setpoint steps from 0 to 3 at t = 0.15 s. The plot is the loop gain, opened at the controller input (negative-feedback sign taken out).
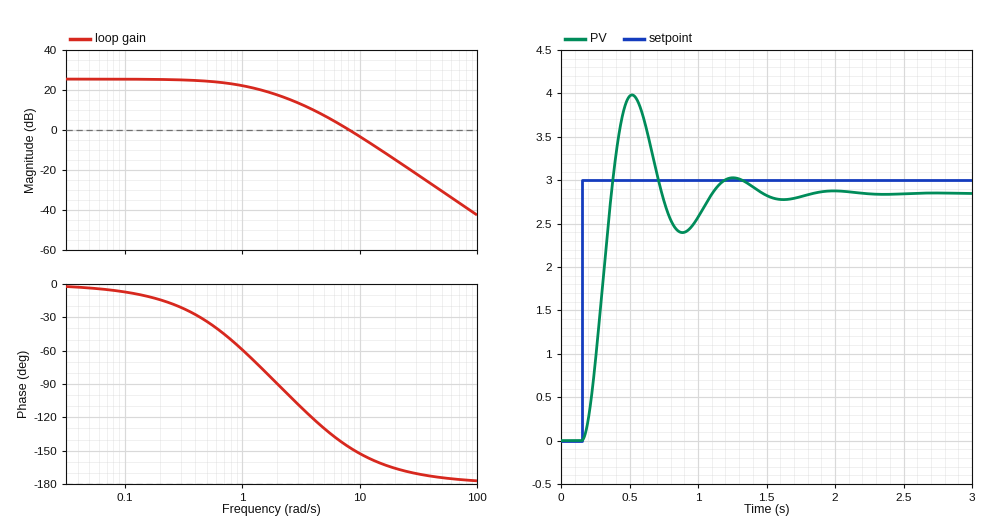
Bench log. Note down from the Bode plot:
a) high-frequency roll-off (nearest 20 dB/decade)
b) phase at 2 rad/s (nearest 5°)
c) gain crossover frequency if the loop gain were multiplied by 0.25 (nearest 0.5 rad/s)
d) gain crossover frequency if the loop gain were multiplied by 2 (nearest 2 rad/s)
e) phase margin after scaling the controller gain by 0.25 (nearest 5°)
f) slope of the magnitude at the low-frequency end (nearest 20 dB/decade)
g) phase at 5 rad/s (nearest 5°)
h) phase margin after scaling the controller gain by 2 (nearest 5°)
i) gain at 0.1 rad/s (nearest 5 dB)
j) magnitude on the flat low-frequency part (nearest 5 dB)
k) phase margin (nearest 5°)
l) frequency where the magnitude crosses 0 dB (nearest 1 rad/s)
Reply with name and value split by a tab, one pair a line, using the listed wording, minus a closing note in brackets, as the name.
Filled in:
high-frequency roll-off	-40 dB/decade
phase at 2 rad/s	-90°
gain crossover frequency if the loop gain were multiplied by 0.25	3.5 rad/s
gain crossover frequency if the loop gain were multiplied by 2	12 rad/s
phase margin after scaling the controller gain by 0.25	65°
slope of the magnitude at the low-frequency end	0 dB/decade
phase at 5 rad/s	-130°
phase margin after scaling the controller gain by 2	25°
gain at 0.1 rad/s	25 dB
magnitude on the flat low-frequency part	25 dB
phase margin	35°
frequency where the magnitude crosses 0 dB	8 rad/s
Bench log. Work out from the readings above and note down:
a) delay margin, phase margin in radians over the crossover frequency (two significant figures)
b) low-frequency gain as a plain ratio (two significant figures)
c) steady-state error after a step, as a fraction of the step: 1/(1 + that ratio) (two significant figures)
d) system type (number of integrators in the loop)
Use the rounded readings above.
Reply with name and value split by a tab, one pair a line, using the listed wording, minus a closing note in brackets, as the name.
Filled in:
delay margin, phase margin in radians over the crossover frequency	0.076 s
low-frequency gain as a plain ratio	18
steady-state error after a step, as a fraction of the step: 1/(1 + that ratio)	0.053
system type	0
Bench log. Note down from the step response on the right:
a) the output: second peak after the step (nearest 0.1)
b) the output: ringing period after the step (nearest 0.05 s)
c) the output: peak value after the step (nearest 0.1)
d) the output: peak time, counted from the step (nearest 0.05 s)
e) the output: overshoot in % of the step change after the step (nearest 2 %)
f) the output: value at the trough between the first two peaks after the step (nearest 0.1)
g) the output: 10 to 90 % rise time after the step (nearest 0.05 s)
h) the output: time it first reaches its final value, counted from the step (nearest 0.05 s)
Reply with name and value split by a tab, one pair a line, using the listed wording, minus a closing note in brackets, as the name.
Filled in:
the output: second peak after the step	3.0
the output: ringing period after the step	0.75 s
the output: peak value after the step	4.0
the output: peak time, counted from the step	0.35 s
the output: overshoot in % of the step change after the step	40 %
the output: value at the trough between the first two peaks after the step	2.4
the output: 10 to 90 % rise time after the step	0.15 s
the output: time it first reaches its final value, counted from the step	0.20 s
